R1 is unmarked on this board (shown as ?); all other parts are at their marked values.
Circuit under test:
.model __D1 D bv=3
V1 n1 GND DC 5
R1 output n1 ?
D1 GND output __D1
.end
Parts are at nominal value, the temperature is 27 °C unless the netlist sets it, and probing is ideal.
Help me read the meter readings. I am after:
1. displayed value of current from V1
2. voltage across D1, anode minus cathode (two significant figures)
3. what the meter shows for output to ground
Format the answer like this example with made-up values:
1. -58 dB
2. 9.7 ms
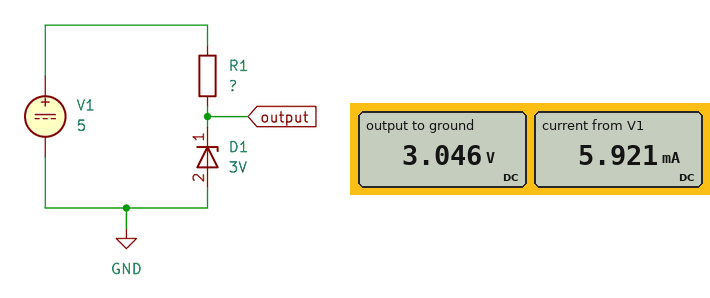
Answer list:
1. 5.921 mA
2. -3.0 V
3. 3.046 V
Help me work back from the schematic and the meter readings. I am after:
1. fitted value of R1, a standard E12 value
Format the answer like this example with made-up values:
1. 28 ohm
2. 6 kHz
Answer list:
1. 330 Ω
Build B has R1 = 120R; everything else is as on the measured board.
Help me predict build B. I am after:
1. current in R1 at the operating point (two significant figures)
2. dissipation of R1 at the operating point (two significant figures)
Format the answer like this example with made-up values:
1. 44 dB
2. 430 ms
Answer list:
1. 16 mA
2. 31 mW
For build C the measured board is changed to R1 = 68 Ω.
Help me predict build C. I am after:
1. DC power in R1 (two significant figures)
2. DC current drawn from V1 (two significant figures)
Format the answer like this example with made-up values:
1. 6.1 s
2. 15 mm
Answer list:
1. 54 mW
2. 28 mA
